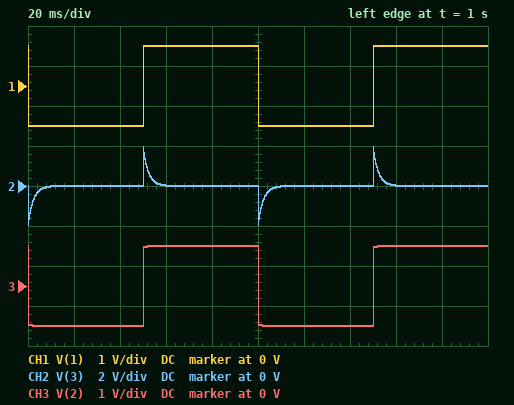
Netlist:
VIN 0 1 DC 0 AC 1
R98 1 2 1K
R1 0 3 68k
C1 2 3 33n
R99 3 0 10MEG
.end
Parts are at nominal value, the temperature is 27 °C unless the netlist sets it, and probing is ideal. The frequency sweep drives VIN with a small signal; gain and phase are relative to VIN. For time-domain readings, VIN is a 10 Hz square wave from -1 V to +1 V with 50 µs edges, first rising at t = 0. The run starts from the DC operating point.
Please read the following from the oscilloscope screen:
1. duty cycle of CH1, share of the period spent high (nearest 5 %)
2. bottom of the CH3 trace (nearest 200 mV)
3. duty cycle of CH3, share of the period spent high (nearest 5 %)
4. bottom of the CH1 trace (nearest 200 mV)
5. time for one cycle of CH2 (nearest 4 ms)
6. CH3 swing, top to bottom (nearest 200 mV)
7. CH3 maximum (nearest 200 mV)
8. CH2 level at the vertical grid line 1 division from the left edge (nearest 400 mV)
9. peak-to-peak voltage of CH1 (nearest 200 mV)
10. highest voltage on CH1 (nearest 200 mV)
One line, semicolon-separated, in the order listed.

50 %; -1.0 V; 50 %; -1.0 V; 100 ms; 2.0 V; 1.0 V; 0 V; 2.0 V; 1.0 V
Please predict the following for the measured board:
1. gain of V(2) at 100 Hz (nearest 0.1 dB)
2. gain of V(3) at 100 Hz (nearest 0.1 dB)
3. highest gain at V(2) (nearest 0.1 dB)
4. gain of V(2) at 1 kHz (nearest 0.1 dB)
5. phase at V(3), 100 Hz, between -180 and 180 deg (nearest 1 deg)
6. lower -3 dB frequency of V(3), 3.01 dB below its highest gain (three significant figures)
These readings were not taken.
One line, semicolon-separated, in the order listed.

-0.1 dB; -1.9 dB; 0 dB; -0.1 dB; -145 deg; 70.4 Hz
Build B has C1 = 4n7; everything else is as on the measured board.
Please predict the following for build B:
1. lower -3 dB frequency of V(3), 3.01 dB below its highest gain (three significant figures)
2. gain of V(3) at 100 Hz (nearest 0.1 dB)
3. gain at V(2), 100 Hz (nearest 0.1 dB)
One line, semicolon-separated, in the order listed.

494 Hz; -14.2 dB; 0 dB
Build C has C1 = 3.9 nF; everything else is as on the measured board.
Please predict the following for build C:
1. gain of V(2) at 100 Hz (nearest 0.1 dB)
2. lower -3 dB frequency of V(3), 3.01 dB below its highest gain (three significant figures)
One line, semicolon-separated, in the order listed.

0 dB; 595 Hz
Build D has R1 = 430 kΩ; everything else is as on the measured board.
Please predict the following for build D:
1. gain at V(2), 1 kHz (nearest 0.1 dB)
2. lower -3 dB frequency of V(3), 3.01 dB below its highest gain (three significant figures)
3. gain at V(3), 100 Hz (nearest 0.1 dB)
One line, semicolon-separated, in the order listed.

0 dB; 11.7 Hz; -0.1 dB
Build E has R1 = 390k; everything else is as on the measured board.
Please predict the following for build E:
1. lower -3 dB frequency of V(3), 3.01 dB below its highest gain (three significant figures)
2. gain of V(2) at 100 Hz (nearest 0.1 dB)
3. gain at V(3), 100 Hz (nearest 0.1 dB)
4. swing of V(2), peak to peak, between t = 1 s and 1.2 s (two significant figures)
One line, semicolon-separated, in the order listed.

12.8 Hz; 0 dB; -0.1 dB; 2.0 V
